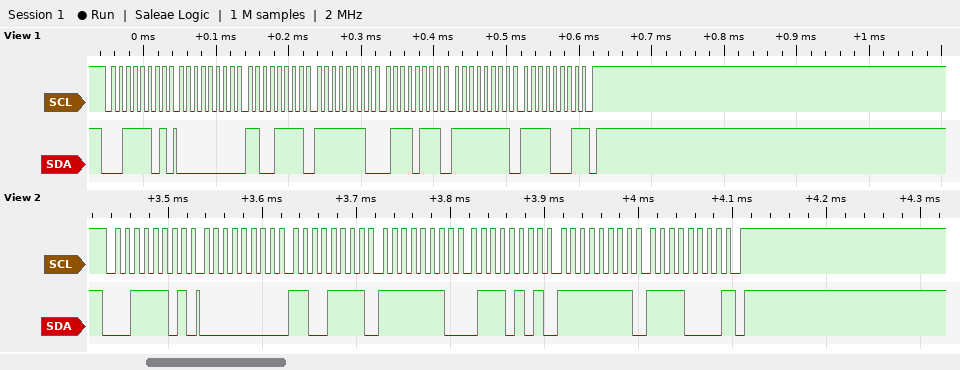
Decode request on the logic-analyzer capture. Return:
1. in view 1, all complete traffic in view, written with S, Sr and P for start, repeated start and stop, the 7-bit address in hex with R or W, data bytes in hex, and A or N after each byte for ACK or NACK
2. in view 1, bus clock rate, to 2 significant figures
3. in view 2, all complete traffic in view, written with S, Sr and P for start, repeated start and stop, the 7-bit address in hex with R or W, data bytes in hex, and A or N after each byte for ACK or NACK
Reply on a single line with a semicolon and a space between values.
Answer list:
S 1ER A 00 A CF A FE A 77 A FF A F1 N P; 100 kHz; S 1ER A 00 A CF A FE A 75 A FF A F0 N P
